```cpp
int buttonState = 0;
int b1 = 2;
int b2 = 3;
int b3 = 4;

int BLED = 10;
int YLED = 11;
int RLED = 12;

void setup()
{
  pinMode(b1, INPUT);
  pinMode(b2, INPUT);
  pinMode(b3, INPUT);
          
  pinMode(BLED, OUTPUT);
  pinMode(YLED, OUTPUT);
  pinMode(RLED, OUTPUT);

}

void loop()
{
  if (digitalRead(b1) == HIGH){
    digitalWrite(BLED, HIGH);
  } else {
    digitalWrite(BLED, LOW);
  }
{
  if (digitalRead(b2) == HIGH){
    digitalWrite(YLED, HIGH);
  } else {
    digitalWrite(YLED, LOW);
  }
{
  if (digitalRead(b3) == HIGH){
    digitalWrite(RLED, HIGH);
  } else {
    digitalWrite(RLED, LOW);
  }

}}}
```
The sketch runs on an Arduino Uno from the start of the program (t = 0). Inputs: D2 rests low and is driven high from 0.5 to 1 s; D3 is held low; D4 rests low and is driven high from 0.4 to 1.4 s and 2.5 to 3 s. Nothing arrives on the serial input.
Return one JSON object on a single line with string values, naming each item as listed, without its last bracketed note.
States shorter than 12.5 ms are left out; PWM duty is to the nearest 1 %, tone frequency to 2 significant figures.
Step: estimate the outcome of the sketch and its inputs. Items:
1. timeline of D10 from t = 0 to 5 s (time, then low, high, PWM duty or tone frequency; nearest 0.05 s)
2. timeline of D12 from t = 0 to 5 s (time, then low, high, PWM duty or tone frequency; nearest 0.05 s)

{"timeline of D10 from t = 0 to 5 s": "0 s low; 0.5 s high; 1 s low", "timeline of D12 from t = 0 to 5 s": "0 s low; 0.4 s high; 1.4 s low; 2.5 s high; 3 s low"}
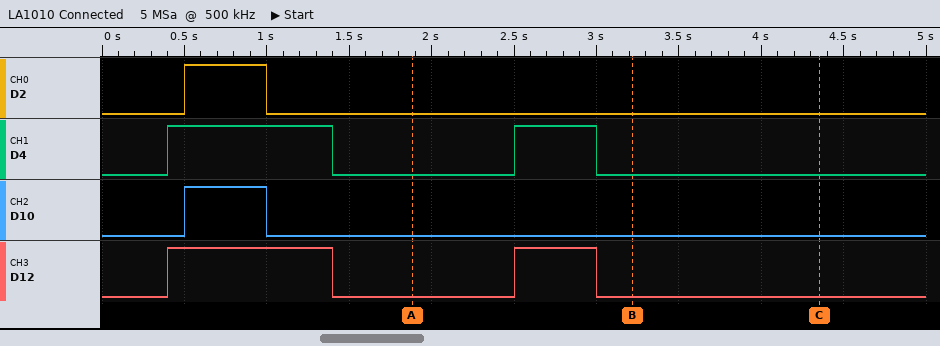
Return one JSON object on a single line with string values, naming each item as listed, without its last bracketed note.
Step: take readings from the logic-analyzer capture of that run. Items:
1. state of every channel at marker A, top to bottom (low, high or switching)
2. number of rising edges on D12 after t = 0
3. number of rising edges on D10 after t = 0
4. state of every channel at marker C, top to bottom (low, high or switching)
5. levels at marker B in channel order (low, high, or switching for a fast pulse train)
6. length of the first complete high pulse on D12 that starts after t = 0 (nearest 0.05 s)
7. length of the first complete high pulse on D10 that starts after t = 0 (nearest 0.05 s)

{"state of every channel at marker A, top to bottom": "D2 low, D4 low, D10 low, D12 low", "number of rising edges on D12 after t = 0": "2", "number of rising edges on D10 after t = 0": "1", "state of every channel at marker C, top to bottom": "D2 low, D4 low, D10 low, D12 low", "levels at marker B in channel order": "D2 low, D4 low, D10 low, D12 low", "length of the first complete high pulse on D12 that starts after t = 0": "1.00 s", "length of the first complete high pulse on D10 that starts after t = 0": "0.50 s"}
